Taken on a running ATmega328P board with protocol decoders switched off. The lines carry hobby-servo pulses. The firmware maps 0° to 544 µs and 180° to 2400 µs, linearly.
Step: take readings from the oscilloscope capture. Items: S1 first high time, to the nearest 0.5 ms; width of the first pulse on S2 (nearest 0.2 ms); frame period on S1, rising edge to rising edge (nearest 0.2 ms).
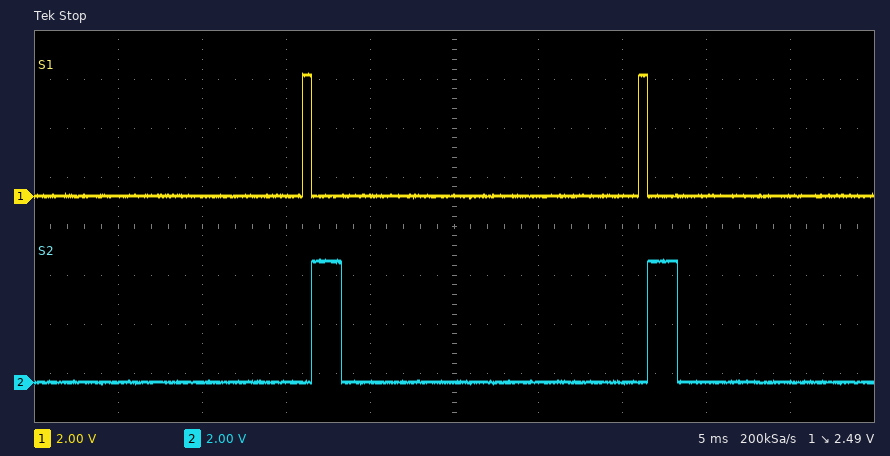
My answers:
0.5 ms
1.8 ms
20.0 ms
